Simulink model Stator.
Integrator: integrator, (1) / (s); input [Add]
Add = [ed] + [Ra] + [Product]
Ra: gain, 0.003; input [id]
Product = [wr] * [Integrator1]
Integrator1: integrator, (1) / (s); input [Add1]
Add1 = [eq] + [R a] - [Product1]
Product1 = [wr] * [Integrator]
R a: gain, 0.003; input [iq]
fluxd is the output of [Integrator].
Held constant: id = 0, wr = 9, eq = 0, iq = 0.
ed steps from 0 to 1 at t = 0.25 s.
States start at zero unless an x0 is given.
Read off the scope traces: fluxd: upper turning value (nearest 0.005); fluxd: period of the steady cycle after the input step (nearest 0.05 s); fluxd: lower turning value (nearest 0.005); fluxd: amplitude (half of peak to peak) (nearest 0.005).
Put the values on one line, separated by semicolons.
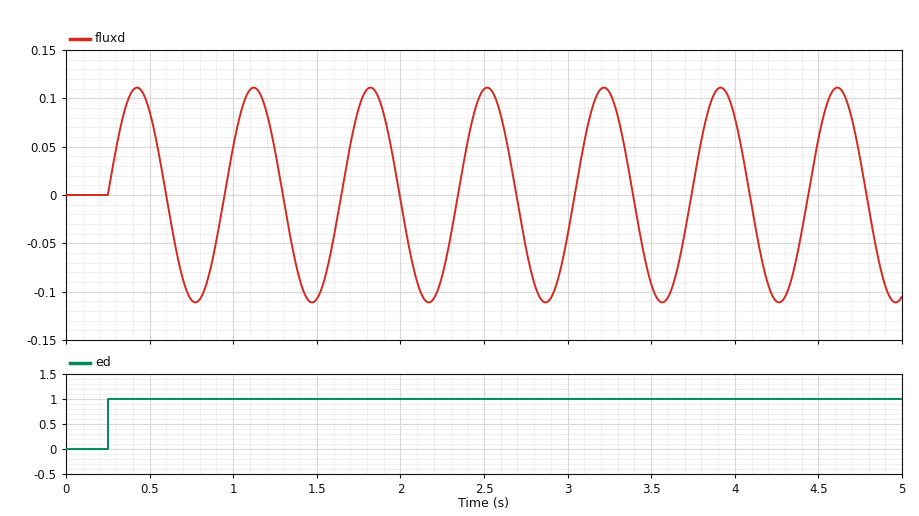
0.110; 0.70 s; -0.110; 0.110
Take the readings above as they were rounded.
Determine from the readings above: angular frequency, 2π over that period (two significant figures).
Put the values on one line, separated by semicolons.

9.0 rad/s
